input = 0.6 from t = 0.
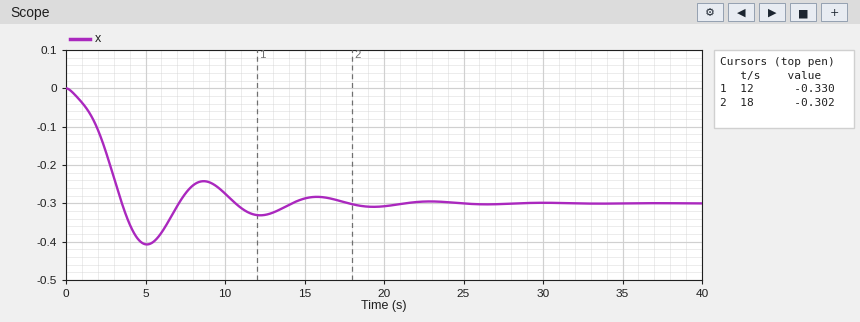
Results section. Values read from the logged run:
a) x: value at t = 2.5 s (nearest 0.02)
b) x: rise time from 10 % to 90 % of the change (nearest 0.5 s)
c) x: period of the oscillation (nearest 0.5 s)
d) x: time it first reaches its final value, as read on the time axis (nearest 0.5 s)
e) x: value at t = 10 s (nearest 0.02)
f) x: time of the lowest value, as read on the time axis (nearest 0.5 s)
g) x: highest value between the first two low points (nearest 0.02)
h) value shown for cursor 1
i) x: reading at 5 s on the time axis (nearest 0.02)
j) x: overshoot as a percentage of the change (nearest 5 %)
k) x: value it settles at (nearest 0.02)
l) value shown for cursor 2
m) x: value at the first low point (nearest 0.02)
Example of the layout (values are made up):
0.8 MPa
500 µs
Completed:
-0.16
2.5 s
7.0 s
3.5 s
-0.28
5.0 s
-0.24
-0.330
-0.40
35 %
-0.30
-0.302
-0.40
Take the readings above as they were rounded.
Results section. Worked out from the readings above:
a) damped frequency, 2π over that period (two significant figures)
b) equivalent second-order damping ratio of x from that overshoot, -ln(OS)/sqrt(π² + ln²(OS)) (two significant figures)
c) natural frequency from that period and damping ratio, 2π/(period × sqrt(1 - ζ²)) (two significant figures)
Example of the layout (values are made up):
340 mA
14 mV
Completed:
0.90 rad/s
0.32
0.95 rad/s
